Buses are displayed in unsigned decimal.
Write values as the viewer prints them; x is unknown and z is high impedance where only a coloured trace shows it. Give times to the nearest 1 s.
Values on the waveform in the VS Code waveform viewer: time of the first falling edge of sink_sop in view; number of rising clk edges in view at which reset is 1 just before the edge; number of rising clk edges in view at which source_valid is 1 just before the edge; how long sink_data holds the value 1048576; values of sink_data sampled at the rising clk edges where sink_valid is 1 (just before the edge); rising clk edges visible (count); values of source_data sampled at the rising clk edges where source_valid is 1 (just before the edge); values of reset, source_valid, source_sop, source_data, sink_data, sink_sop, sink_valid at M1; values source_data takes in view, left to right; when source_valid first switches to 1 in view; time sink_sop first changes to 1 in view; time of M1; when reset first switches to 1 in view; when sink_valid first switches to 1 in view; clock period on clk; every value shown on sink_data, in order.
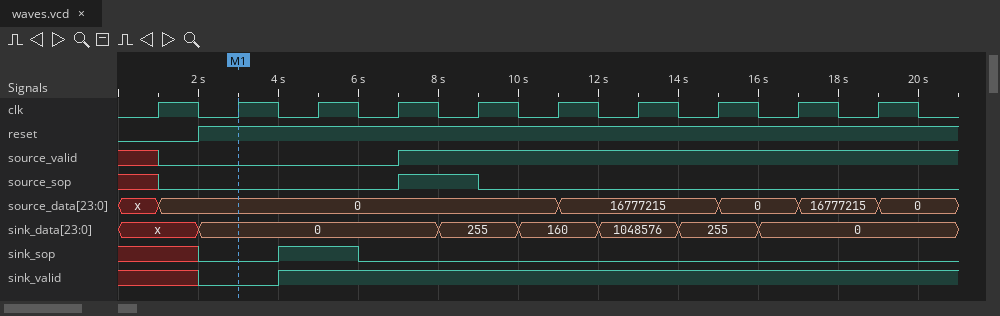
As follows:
6 s
9
6
2 s
0, 0, 255, 160, 1048576, 255, 0, 0
10
0, 0, 16777215, 16777215, 0, 16777215
reset=1, source_valid=0, source_sop=0, source_data=0, sink_data=0, sink_sop=0, sink_valid=0
x, 0, 16777215, 0, 16777215, 0
7 s
4 s
3 s
2 s
4 s
2 s
x, 0, 255, 160, 1048576, 255, 0
